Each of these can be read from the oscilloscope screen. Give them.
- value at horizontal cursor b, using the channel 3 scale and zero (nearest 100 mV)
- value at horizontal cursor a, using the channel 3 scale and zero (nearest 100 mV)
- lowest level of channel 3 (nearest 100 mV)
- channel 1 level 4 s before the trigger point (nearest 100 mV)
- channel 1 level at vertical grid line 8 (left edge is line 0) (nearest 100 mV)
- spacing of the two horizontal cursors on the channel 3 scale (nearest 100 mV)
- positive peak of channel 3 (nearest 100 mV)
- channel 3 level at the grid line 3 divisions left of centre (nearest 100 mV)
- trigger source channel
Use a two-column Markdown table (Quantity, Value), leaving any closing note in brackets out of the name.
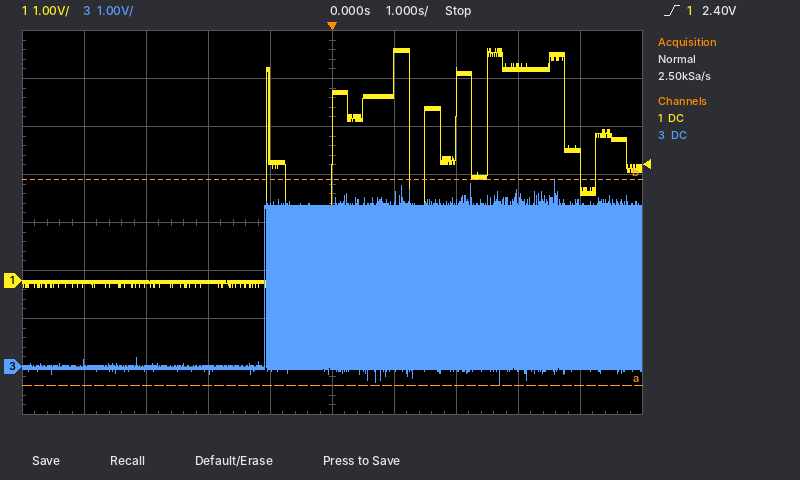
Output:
| Quantity | Value |
|---|---|
| value at horizontal cursor b, using the channel 3 scale and zero | 3.9 V |
| value at horizontal cursor a, using the channel 3 scale and zero | -400 mV |
| lowest level of channel 3 | -400 mV |
| channel 1 level 4 s before the trigger point | -100 mV |
| channel 1 level at vertical grid line 8 (left edge is line 0) | 4.4 V |
| spacing of the two horizontal cursors on the channel 3 scale | 4.3 V |
| positive peak of channel 3 | 3.9 V |
| channel 3 level at the grid line 3 divisions left of centre | 0.0 V |
| trigger source channel | channel 1 |
